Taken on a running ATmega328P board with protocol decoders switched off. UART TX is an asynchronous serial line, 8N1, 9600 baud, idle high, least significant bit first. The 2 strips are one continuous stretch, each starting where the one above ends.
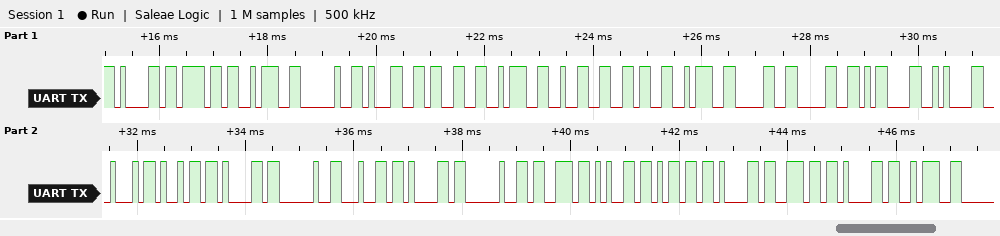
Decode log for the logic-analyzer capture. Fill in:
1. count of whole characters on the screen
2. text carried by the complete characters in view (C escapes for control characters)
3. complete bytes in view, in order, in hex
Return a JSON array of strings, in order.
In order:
["28", "\"ao: 13:26:00\\r\\nDia da semana:\"", "61 6F 3A 20 31 33 3A 32 36 3A 30 30 0D 0A 44 69 61 20 64 61 20 73 65 6D 61 6E 61 3A"]
